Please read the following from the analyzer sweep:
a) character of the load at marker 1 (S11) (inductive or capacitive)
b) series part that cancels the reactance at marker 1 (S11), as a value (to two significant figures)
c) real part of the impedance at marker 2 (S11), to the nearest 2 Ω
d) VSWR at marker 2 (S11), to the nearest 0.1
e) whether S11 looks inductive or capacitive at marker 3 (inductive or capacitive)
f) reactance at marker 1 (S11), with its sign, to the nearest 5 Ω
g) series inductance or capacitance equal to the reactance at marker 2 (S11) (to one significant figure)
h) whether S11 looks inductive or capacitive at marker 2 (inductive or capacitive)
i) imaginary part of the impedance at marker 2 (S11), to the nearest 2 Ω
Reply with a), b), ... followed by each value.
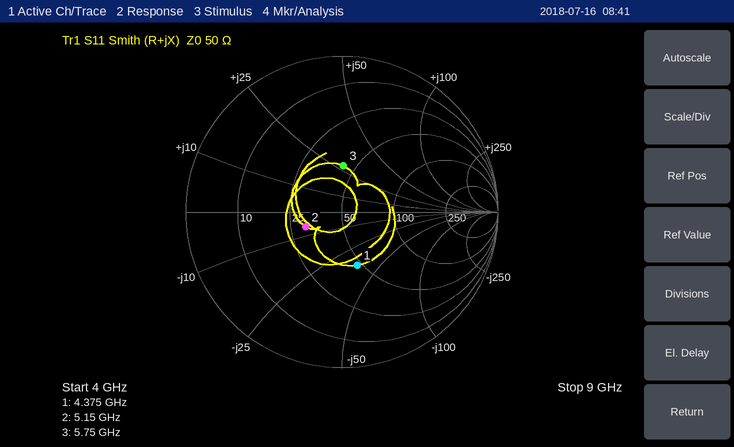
a) capacitive
b) 1.3 nH
c) 30 Ω
d) 1.7
e) inductive
f) -35 Ω
g) 5 pF
h) capacitive
i) -6 Ω
